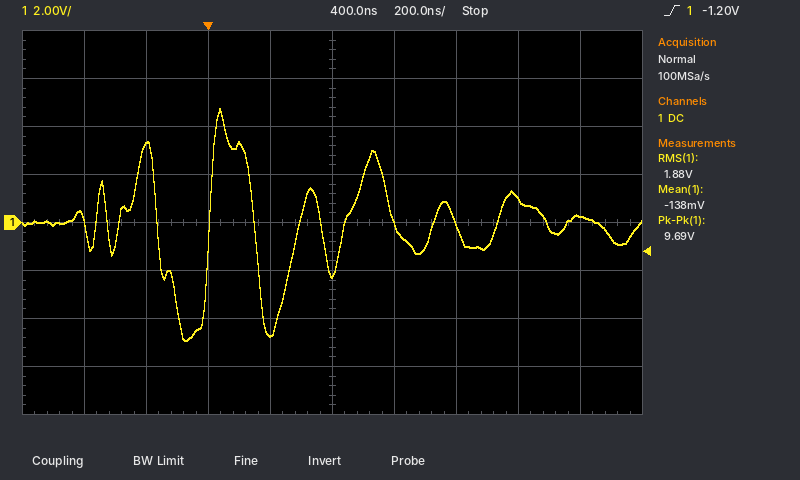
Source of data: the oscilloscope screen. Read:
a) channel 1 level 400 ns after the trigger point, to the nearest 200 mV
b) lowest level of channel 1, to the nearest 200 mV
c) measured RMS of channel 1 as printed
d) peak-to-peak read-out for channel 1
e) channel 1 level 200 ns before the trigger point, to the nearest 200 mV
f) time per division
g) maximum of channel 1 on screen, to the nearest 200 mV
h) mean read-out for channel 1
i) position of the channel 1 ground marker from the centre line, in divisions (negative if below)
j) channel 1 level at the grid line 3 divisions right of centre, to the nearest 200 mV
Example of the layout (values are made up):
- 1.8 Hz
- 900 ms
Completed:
- -2.2 V
- -5.0 V
- 1.88 V
- 9.69 V
- 3.2 V
- 200 ns
- 4.8 V
- -138 mV
- 0.0 div
- 1.0 V
